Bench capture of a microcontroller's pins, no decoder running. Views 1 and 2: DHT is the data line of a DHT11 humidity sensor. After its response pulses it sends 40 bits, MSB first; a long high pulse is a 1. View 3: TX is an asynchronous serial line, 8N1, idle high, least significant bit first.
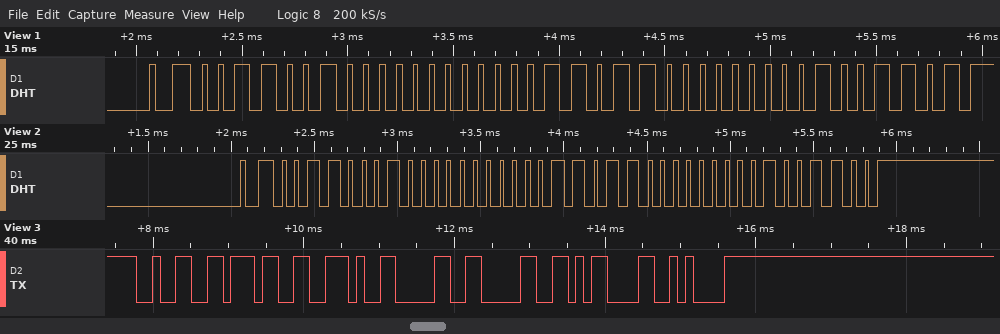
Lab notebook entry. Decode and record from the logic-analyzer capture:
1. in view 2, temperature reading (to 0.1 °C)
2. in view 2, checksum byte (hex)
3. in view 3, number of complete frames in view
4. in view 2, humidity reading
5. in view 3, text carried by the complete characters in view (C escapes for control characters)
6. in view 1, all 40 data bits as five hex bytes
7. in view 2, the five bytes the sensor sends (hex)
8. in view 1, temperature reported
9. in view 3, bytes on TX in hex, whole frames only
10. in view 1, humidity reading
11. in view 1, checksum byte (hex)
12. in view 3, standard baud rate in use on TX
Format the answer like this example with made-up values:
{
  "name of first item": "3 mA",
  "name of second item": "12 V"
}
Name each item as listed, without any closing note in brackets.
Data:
{
  "in view 2, temperature reading": "27.0 °C",
  "in view 2, checksum byte": "0x4C",
  "in view 3, number of complete frames in view": "7",
  "in view 2, humidity reading": "49 %",
  "in view 3, text carried by the complete characters in view": "\"27.00\\r\\n\"",
  "in view 1, all 40 data bits as five hex bytes": "32 00 1B 00 4D",
  "in view 2, the five bytes the sensor sends": "31 00 1B 00 4C",
  "in view 1, temperature reported": "27.0 °C",
  "in view 3, bytes on TX in hex, whole frames only": "0x32 0x37 0x2E 0x30 0x30 0x0D 0x0A",
  "in view 1, humidity reading": "50 %",
  "in view 1, checksum byte": "0x4D",
  "in view 3, standard baud rate in use on TX": "9600 baud"
}
